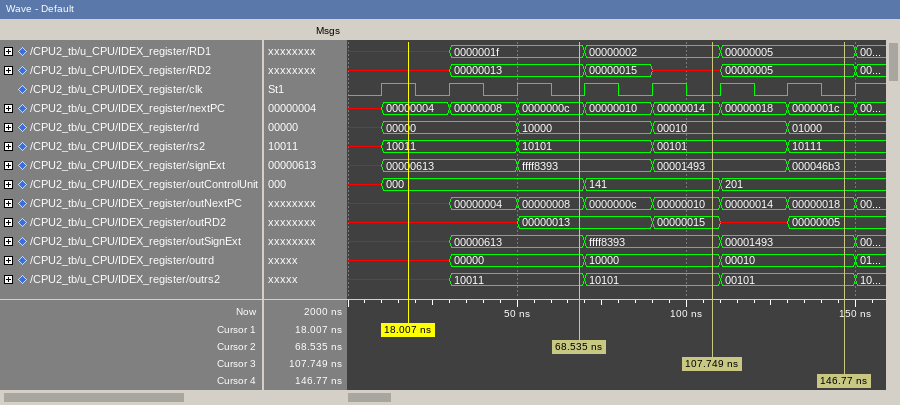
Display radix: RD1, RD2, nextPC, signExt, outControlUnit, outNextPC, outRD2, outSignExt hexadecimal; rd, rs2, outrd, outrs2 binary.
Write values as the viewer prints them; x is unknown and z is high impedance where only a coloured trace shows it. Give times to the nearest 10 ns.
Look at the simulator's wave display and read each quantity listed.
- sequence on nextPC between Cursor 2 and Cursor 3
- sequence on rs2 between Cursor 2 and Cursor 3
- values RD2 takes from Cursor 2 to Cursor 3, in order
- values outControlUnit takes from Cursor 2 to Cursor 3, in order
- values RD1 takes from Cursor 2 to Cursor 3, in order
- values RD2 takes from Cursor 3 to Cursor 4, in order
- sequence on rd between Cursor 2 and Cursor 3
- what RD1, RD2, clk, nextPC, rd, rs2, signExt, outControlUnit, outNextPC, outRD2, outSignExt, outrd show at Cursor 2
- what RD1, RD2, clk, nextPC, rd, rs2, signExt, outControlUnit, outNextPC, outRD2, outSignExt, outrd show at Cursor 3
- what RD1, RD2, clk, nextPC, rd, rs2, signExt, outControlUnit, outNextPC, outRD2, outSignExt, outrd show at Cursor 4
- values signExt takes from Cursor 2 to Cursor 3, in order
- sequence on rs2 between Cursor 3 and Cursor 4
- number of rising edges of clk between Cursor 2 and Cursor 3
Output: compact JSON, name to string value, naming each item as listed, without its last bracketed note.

{"sequence on nextPC between Cursor 2 and Cursor 3": "0000000c, 00000010, 00000014", "sequence on rs2 between Cursor 2 and Cursor 3": "10101, 00101", "values RD2 takes from Cursor 2 to Cursor 3, in order": "00000013, 00000015, x", "values outControlUnit takes from Cursor 2 to Cursor 3, in order": "000, 141", "values RD1 takes from Cursor 2 to Cursor 3, in order": "0000001f, 00000002", "values RD2 takes from Cursor 3 to Cursor 4, in order": "x, 00000005", "sequence on rd between Cursor 2 and Cursor 3": "10000, 00010", "what RD1, RD2, clk, nextPC, rd, rs2, signExt, outControlUnit, outNextPC, outRD2, outSignExt, outrd show at Cursor 2": "RD1=0000001f, RD2=00000013, clk=0, nextPC=0000000c, rd=10000, rs2=10101, signExt=ffff8393, outControlUnit=000, outNextPC=00000008, outRD2=00000013, outSignExt=00000613, outrd=00000", "what RD1, RD2, clk, nextPC, rd, rs2, signExt, outControlUnit, outNextPC, outRD2, outSignExt, outrd show at Cursor 3": "RD1=00000002, RD2=x, clk=0, nextPC=00000014, rd=00010, rs2=00101, signExt=00001493, outControlUnit=141, outNextPC=00000010, outRD2=00000015, outSignExt=ffff8393, outrd=10000", "what RD1, RD2, clk, nextPC, rd, rs2, signExt, outControlUnit, outNextPC, outRD2, outSignExt, outrd show at Cursor 4": "RD1=00000005, RD2=00000005, clk=0, nextPC=0000001c, rd=01000, rs2=10111, signExt=000046b3, outControlUnit=201, outNextPC=00000018, outRD2=00000005, outSignExt=00001493, outrd=00010", "values signExt takes from Cursor 2 to Cursor 3, in order": "ffff8393, 00001493", "sequence on rs2 between Cursor 3 and Cursor 4": "00101, 10111", "number of rising edges of clk between Cursor 2 and Cursor 3": "2"}
